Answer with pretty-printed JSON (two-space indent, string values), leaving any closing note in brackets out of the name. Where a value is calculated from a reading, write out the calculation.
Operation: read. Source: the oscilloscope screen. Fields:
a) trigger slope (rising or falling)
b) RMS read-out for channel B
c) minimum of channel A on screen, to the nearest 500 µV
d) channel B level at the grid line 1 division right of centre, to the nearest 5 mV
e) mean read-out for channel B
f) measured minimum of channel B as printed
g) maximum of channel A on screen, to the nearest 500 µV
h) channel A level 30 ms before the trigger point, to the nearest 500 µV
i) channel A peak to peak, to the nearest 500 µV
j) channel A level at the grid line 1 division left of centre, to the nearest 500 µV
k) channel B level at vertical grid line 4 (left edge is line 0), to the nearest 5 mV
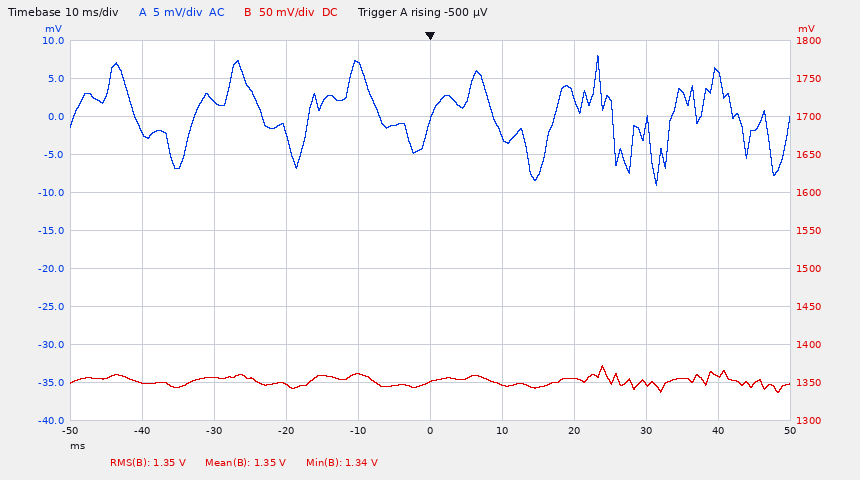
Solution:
{
  "trigger slope": "rising",
  "RMS read-out for channel B": "1.35 V",
  "minimum of channel A on screen, to the nearest 500 µV": "-9.0 mV",
  "channel B level at the grid line 1 division right of centre, to the nearest 5 mV": "1.345 V",
  "mean read-out for channel B": "1.35 V",
  "measured minimum of channel B as printed": "1.34 V",
  "maximum of channel A on screen, to the nearest 500 µV": "8.0 mV",
  "channel A level 30 ms before the trigger point, to the nearest 500 µV": "2.0 mV",
  "channel A peak to peak, to the nearest 500 µV": "8.0 mV − (-9.0 mV) = 17.0 mV",
  "channel A level at the grid line 1 division left of centre, to the nearest 500 µV": "7.0 mV",
  "channel B level at vertical grid line 4 (left edge is line 0), to the nearest 5 mV": "1.360 V"
}
